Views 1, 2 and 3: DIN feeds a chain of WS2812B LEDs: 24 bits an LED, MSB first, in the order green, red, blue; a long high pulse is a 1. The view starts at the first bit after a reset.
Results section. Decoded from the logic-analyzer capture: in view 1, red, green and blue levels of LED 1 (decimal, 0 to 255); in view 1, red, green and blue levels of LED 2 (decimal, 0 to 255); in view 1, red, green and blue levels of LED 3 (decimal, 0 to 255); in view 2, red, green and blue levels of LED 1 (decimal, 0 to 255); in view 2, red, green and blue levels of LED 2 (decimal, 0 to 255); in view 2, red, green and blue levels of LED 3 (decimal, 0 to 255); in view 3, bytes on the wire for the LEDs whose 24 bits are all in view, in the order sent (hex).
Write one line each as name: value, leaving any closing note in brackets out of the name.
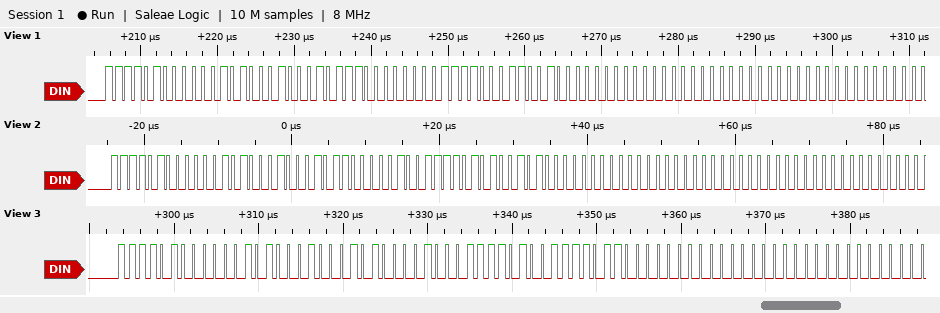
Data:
in view 1, red, green and blue levels of LED 1: 10, 244, 34
in view 1, red, green and blue levels of LED 2: 30, 224, 50
in view 1, red, green and blue levels of LED 3: 0, 0, 0
in view 2, red, green and blue levels of LED 1: 10, 244, 34
in view 2, red, green and blue levels of LED 2: 61, 193, 74
in view 2, red, green and blue levels of LED 3: 0, 0, 0
in view 3, bytes on the wire for the LEDs whose 24 bits are all in view, in the order sent: F4 0A 22 84 7A 7B 00 00 00
